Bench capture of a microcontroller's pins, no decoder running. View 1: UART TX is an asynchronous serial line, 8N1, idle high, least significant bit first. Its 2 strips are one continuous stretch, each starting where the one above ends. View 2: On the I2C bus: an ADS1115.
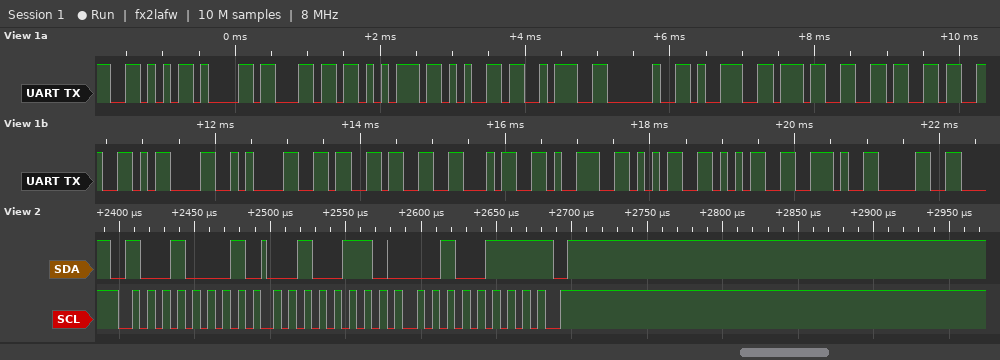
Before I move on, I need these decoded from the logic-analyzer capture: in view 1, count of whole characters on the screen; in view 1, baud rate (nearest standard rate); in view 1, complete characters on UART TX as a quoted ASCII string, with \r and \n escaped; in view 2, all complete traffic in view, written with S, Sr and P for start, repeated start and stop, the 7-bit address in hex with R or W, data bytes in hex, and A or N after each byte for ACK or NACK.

21
9600 baud
"Value: 9763\r\n634955.0"
S 48R A 26 A 27 N P
